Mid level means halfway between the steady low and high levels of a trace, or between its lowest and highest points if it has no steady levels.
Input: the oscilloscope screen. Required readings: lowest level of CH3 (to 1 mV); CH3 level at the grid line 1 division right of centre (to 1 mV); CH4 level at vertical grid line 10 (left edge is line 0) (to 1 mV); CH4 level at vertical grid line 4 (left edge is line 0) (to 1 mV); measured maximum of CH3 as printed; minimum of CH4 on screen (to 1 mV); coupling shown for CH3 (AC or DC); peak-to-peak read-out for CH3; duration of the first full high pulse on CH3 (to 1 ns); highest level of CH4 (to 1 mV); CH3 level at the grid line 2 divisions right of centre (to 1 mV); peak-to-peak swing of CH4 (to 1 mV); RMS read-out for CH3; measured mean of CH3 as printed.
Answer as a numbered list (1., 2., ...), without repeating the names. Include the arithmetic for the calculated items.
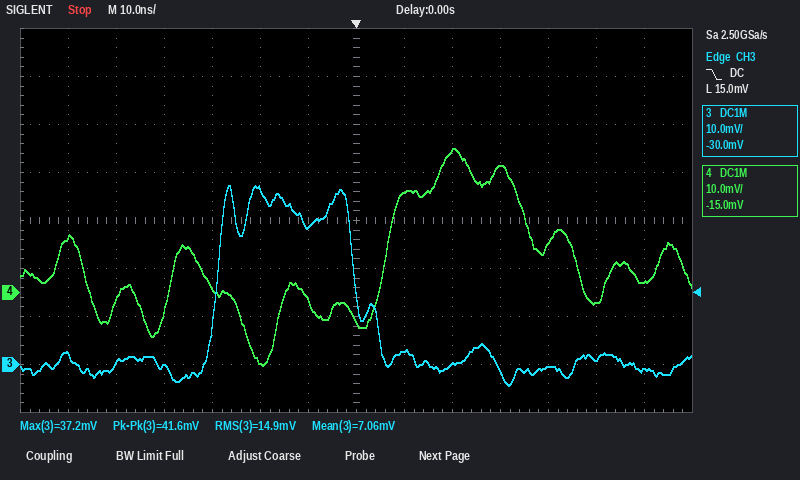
1. -4 mV
2. 3 mV
3. 26 mV
4. 1 mV
5. 37.2 mV
6. -15 mV
7. DC
8. 41.6 mV
9. 29 ns
10. 30 mV
11. 0 mV
12. 30 mV − (-15 mV) = 45 mV
13. 14.9 mV
14. 7.06 mV
